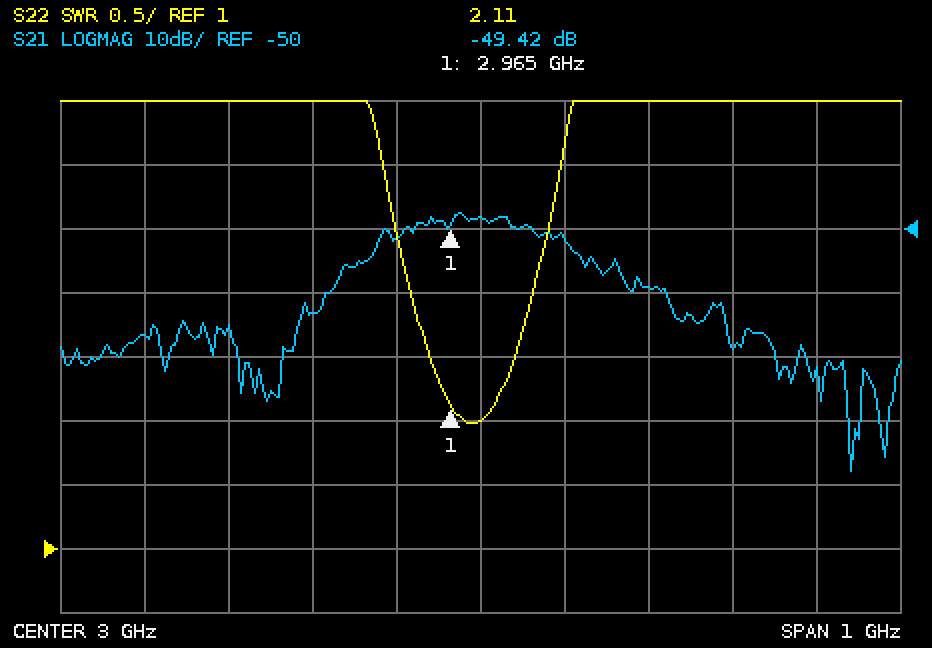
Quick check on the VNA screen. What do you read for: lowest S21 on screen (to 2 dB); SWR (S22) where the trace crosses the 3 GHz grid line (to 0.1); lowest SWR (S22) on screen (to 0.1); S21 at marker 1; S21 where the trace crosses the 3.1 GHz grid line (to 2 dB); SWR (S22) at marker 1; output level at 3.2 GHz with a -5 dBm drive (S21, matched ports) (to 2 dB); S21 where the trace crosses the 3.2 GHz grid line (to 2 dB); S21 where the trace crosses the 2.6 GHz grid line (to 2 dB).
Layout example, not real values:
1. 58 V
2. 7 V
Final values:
1. -88 dB
2. 2.0
3. 2.0
4. -49.42 dB
5. -52 dB
6. 2.11
7. -64 dBm
8. -60 dB
9. -66 dB
